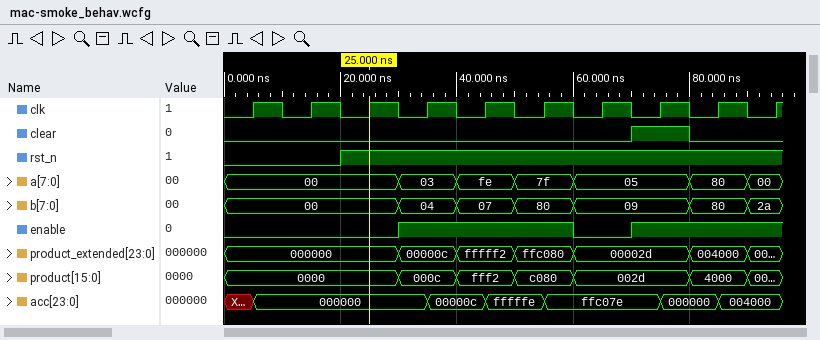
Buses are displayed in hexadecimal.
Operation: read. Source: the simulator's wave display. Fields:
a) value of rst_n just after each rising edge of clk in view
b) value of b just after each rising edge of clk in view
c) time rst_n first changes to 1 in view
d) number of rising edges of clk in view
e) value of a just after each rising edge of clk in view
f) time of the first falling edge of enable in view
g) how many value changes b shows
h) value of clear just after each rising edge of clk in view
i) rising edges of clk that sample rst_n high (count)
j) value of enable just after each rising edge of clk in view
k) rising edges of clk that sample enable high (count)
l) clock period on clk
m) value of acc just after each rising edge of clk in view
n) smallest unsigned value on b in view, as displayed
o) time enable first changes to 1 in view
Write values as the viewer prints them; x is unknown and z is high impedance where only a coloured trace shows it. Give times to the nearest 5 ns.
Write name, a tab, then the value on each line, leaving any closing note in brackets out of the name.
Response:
value of rst_n just after each rising edge of clk in view	0 0 1 1 1 1 1 1 1 1
value of b just after each rising edge of clk in view	00, 00, 00, 04, 07, 80, 09, 09, 80, 2a
time rst_n first changes to 1 in view	20 ns
number of rising edges of clk in view	10
value of a just after each rising edge of clk in view	00, 00, 00, 03, fe, 7f, 05, 05, 80, 00
time of the first falling edge of enable in view	60 ns
how many value changes b shows	6
value of clear just after each rising edge of clk in view	0 0 0 0 0 0 0 1 0 0
rising edges of clk that sample rst_n high	8
value of enable just after each rising edge of clk in view	0 0 0 1 1 1 0 1 1 1
rising edges of clk that sample enable high	6
clock period on clk	10 ns
value of acc just after each rising edge of clk in view	000000, 000000, 000000, 00000c, fffffe, ffc07e, ffc07e, 000000, 004000, 004000
smallest unsigned value on b in view, as displayed	00
time enable first changes to 1 in view	30 ns
